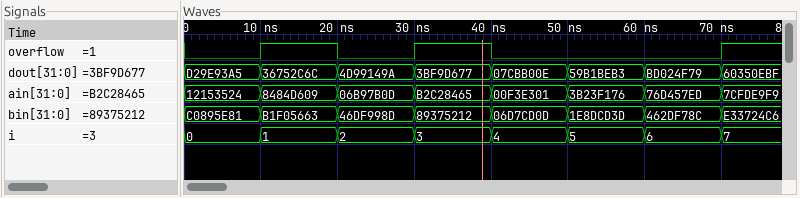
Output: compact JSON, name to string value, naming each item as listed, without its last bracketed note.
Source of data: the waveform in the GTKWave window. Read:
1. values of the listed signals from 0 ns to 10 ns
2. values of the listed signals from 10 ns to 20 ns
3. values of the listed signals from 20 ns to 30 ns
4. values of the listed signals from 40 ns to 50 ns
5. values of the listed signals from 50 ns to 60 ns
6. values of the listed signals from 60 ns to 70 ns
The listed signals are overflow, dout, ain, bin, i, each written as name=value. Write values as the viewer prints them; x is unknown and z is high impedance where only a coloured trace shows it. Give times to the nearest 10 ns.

{"values of the listed signals from 0 ns to 10 ns": "overflow=0, dout=D29E93A5, ain=12153524, bin=C0895E81, i=0", "values of the listed signals from 10 ns to 20 ns": "overflow=1, dout=36752C6C, ain=8484D609, bin=B1F05663, i=1", "values of the listed signals from 20 ns to 30 ns": "overflow=0, dout=4D99149A, ain=06B97B0D, bin=46DF998D, i=2", "values of the listed signals from 40 ns to 50 ns": "overflow=0, dout=07CBB00E, ain=00F3E301, bin=06D7CD0D, i=4", "values of the listed signals from 50 ns to 60 ns": "overflow=0, dout=59B1BEB3, ain=3B23F176, bin=1E8DCD3D, i=5", "values of the listed signals from 60 ns to 70 ns": "overflow=0, dout=BD024F79, ain=76D457ED, bin=462DF78C, i=6"}
